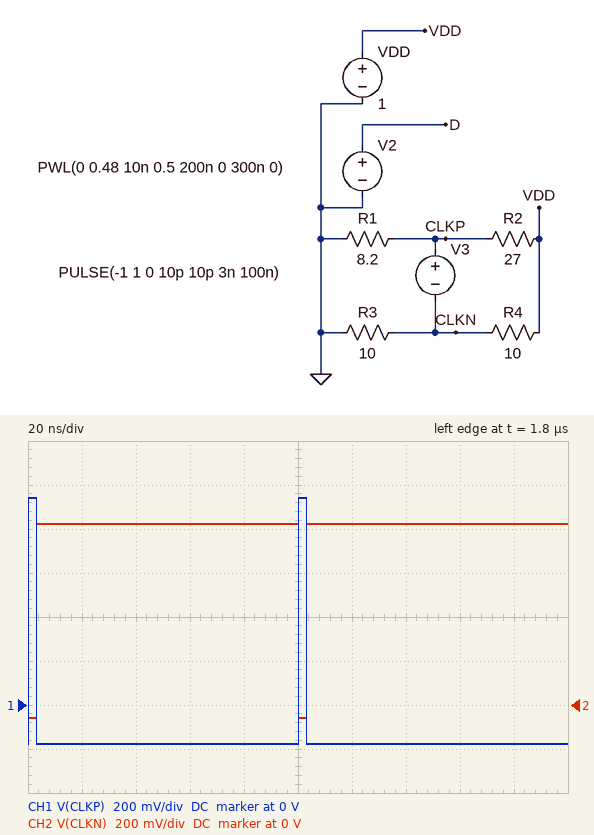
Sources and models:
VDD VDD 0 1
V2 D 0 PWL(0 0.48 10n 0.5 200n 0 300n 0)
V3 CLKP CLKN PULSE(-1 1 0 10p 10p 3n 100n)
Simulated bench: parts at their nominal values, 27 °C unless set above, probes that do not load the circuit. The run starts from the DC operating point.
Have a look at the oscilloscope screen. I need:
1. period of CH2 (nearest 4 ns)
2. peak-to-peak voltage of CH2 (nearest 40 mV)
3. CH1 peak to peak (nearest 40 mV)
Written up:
100 ns
880 mV
1.12 V
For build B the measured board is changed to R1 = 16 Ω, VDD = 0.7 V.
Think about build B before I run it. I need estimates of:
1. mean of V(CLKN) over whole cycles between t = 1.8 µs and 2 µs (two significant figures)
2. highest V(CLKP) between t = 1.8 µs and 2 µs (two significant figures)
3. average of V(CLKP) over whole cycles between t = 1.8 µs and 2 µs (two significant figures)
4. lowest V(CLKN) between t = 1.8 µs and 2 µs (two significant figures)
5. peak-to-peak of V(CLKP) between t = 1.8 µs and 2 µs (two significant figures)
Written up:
630 mV
990 mV
-310 mV
-12 mV
1.3 V
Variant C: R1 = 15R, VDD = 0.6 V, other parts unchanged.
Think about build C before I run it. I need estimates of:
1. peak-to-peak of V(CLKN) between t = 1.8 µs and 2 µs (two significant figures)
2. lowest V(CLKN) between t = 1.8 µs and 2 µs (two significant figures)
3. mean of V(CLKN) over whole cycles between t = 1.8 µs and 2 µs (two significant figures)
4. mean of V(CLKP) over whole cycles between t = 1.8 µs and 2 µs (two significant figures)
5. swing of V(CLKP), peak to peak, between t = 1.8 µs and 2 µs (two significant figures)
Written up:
680 mV
-71 mV
590 mV
-350 mV
1.3 V
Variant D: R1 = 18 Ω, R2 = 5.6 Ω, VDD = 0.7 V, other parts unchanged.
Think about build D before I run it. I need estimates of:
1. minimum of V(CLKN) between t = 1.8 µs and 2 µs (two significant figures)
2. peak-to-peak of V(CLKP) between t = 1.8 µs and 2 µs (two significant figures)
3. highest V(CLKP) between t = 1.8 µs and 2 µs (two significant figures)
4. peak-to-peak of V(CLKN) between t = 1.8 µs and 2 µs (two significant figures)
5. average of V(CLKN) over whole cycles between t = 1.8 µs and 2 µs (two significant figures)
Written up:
-90 mV
920 mV
910 mV
1.1 V
960 mV
